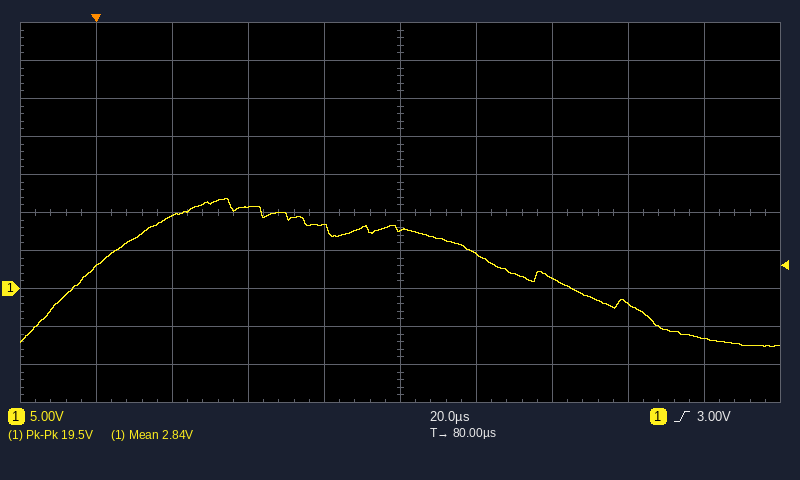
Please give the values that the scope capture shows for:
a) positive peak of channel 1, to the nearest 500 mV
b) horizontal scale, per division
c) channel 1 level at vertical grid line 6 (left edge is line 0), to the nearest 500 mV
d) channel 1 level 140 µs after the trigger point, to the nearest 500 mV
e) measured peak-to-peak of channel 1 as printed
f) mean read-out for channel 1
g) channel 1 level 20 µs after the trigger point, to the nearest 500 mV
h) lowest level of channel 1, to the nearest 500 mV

12.0 V
20 µs
4.5 V
-2.0 V
19.5 V
2.84 V
9.5 V
-7.5 V
